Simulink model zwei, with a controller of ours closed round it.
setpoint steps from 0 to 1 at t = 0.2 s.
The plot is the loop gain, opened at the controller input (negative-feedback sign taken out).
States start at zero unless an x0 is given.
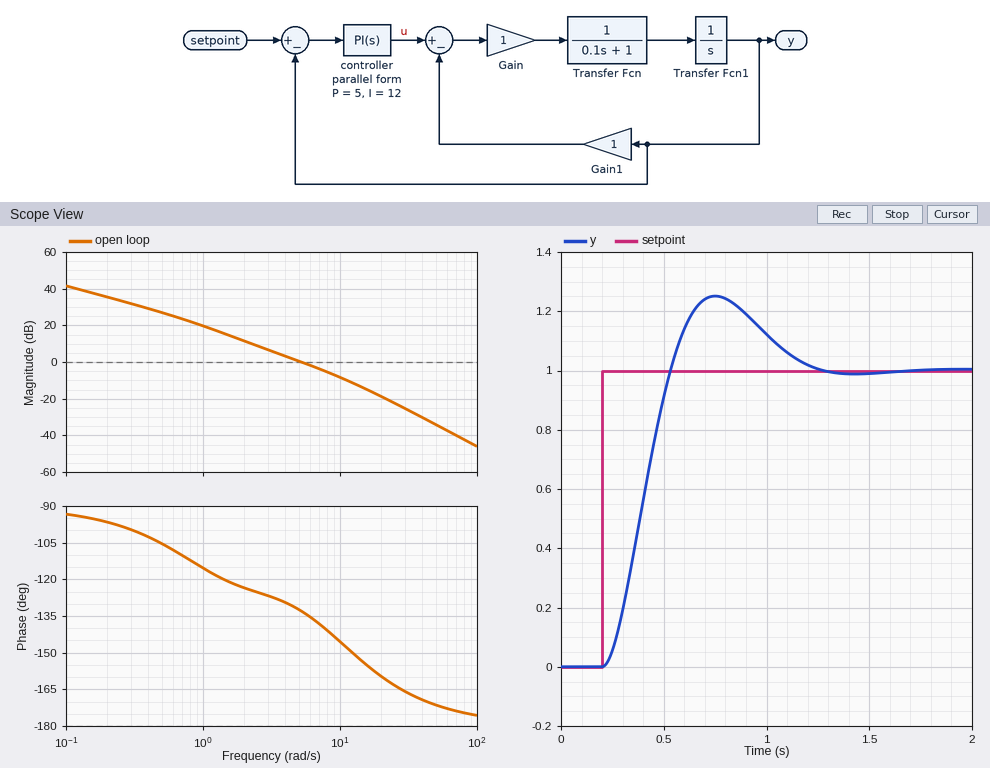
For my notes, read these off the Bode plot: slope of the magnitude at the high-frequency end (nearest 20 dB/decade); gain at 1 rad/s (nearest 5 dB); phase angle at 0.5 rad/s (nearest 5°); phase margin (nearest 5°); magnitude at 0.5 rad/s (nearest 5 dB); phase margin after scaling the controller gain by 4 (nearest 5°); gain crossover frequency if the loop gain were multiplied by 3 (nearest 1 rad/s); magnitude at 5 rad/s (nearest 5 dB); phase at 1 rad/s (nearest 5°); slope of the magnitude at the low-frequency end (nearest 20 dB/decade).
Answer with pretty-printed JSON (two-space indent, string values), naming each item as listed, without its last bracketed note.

{
  "slope of the magnitude at the high-frequency end": "-40 dB/decade",
  "gain at 1 rad/s": "20 dB",
  "phase angle at 0.5 rad/s": "-105°",
  "phase margin": "45°",
  "magnitude at 0.5 rad/s": "25 dB",
  "phase margin after scaling the controller gain by 4": "30°",
  "gain crossover frequency if the loop gain were multiplied by 3": "11 rad/s",
  "magnitude at 5 rad/s": "0 dB",
  "phase at 1 rad/s": "-115°",
  "slope of the magnitude at the low-frequency end": "-20 dB/decade"
}
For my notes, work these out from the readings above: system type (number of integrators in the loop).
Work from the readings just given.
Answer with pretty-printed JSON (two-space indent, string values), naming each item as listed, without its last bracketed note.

{
  "system type": "1"
}
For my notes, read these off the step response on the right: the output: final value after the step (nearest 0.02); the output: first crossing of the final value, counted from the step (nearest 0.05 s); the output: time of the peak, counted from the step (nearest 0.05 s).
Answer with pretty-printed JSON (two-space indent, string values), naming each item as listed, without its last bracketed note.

{
  "the output: final value after the step": "1.00",
  "the output: first crossing of the final value, counted from the step": "0.35 s",
  "the output: time of the peak, counted from the step": "0.55 s"
}
